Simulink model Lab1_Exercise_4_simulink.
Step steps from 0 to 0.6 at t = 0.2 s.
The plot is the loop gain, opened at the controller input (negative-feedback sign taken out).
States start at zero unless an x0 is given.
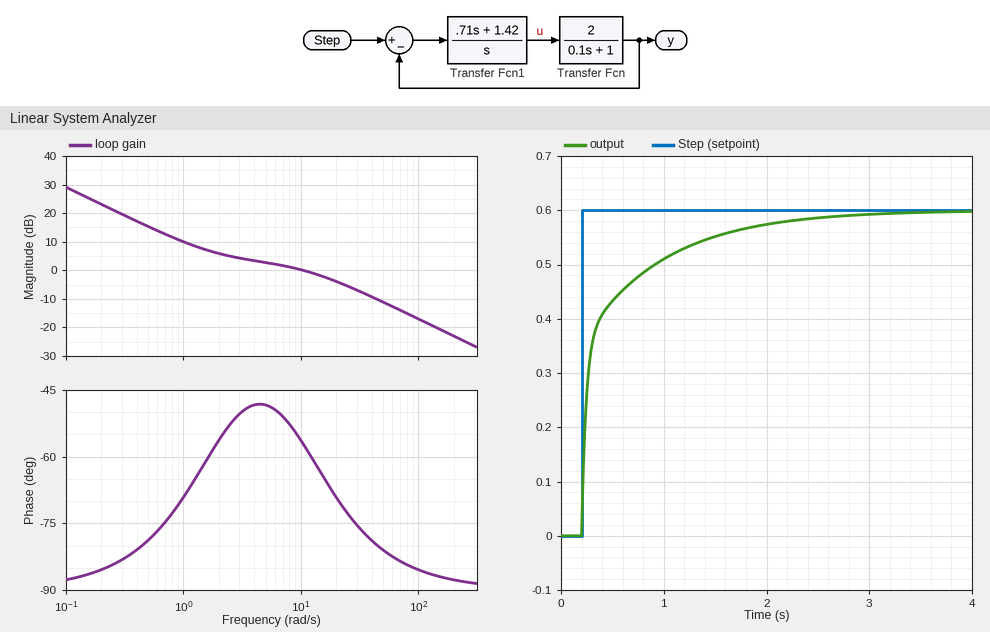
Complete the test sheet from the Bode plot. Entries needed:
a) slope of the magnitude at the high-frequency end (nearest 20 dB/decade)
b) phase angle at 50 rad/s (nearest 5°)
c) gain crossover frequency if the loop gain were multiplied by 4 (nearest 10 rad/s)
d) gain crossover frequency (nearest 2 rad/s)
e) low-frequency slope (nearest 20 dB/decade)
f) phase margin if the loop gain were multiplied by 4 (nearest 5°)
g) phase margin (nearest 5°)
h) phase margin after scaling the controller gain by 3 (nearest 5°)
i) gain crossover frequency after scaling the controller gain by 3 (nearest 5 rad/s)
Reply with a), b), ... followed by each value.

a) -20 dB/decade
b) -80°
c) 60 rad/s
d) 10 rad/s
e) -20 dB/decade
f) 100°
g) 125°
h) 100°
i) 40 rad/s
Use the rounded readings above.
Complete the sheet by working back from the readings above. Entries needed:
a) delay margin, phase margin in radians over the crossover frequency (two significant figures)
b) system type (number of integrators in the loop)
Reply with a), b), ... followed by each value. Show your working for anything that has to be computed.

a) 125 × π / 180 / 10 = 0.22 s
b) 1
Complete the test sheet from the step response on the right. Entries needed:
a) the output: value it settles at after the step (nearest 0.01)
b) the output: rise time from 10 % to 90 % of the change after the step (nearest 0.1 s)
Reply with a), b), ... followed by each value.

a) 0.60
b) 1.1 s
